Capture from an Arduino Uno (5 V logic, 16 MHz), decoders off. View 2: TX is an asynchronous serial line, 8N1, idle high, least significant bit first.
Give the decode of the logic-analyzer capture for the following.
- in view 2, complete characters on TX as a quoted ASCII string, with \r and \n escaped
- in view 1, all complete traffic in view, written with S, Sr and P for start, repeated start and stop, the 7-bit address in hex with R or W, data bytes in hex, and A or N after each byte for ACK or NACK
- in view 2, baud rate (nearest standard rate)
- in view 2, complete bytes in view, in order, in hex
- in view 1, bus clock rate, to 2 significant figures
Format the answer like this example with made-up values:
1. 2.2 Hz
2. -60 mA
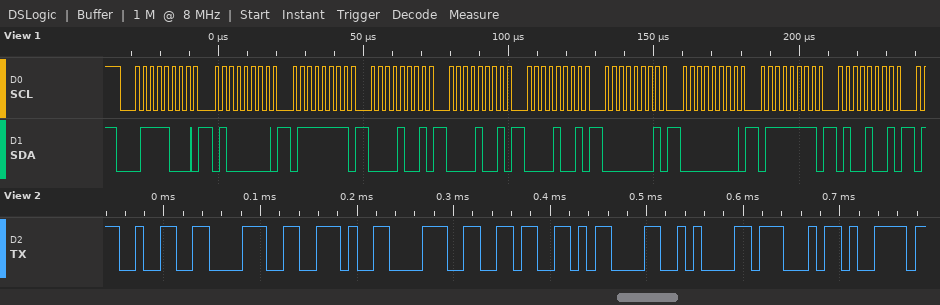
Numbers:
1. "28.86\r\nGy"
2. S 3CW A 40 A 7F A 09 A 09 A 09 A 01 A 00 A 7F A 49 A
3. 115200 baud
4. 32 38 2E 38 36 0D 0A 47 79
5. 400 kHz
